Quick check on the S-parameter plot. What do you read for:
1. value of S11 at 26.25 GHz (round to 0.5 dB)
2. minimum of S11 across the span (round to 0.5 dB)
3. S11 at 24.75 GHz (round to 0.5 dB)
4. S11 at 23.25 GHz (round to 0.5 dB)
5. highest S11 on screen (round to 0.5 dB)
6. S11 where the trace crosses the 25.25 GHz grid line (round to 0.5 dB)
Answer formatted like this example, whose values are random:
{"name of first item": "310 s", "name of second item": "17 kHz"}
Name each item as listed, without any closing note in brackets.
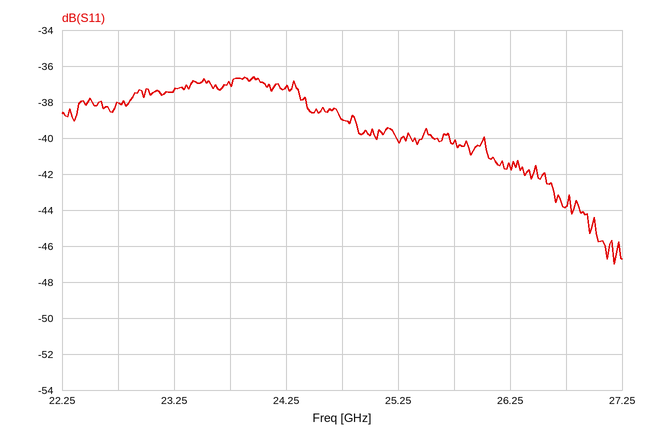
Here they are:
{"value of S11 at 26.25 GHz": "-41.5 dB", "minimum of S11 across the span": "-47.0 dB", "S11 at 24.75 GHz": "-39.0 dB", "S11 at 23.25 GHz": "-37.5 dB", "highest S11 on screen": "-36.5 dB", "S11 where the trace crosses the 25.25 GHz grid line": "-40.0 dB"}
